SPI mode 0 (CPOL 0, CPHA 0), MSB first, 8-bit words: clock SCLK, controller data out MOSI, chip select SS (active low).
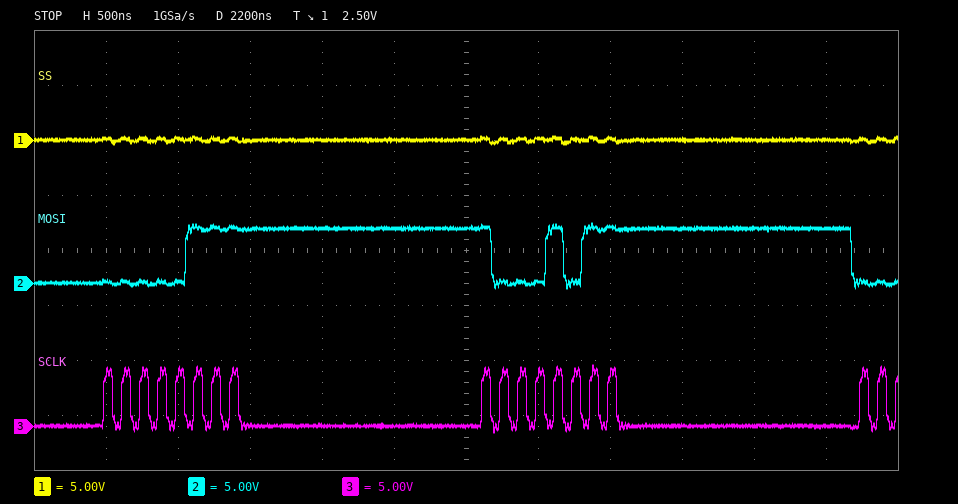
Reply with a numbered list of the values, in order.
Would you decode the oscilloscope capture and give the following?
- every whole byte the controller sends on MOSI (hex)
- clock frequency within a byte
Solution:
1. 0x07 0x8B
2. 8 MHz
